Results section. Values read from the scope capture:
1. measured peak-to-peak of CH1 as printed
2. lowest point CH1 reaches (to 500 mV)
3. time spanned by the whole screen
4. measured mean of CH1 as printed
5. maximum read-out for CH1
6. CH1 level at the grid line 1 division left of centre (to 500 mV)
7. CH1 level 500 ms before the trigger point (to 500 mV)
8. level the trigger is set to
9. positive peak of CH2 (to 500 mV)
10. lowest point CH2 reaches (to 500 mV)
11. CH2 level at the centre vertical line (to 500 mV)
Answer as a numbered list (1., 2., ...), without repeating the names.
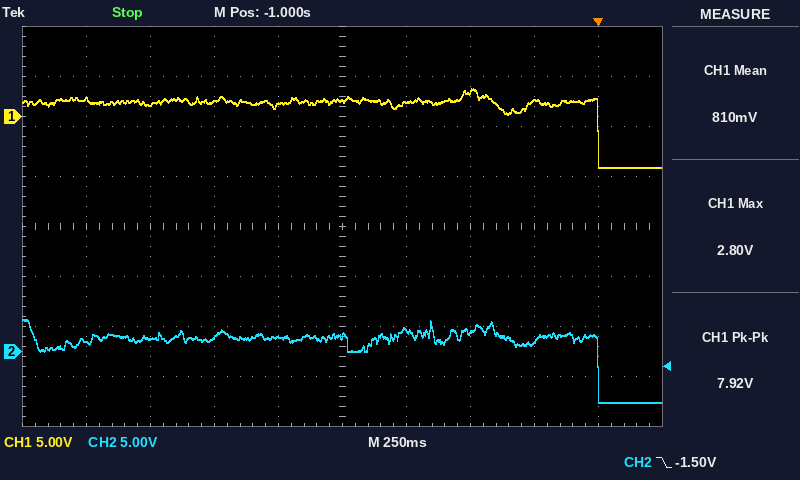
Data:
1. 7.92 V
2. -5.0 V
3. 2.5 s
4. 810 mV
5. 2.80 V
6. 1.0 V
7. 2.5 V
8. -1.50 V
9. 3.0 V
10. -5.0 V
11. 1.5 V
